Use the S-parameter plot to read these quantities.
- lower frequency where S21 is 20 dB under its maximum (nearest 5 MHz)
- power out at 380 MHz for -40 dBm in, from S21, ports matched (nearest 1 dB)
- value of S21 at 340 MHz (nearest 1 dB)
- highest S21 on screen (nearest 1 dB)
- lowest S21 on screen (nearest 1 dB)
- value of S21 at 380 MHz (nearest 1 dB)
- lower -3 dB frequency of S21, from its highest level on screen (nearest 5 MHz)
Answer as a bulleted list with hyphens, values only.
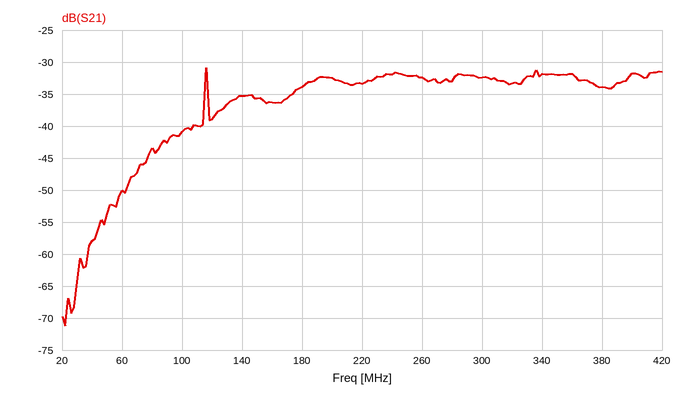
- 60 MHz
- -74 dBm
- -32 dB
- -31 dB
- -71 dB
- -34 dB
- 115 MHz
